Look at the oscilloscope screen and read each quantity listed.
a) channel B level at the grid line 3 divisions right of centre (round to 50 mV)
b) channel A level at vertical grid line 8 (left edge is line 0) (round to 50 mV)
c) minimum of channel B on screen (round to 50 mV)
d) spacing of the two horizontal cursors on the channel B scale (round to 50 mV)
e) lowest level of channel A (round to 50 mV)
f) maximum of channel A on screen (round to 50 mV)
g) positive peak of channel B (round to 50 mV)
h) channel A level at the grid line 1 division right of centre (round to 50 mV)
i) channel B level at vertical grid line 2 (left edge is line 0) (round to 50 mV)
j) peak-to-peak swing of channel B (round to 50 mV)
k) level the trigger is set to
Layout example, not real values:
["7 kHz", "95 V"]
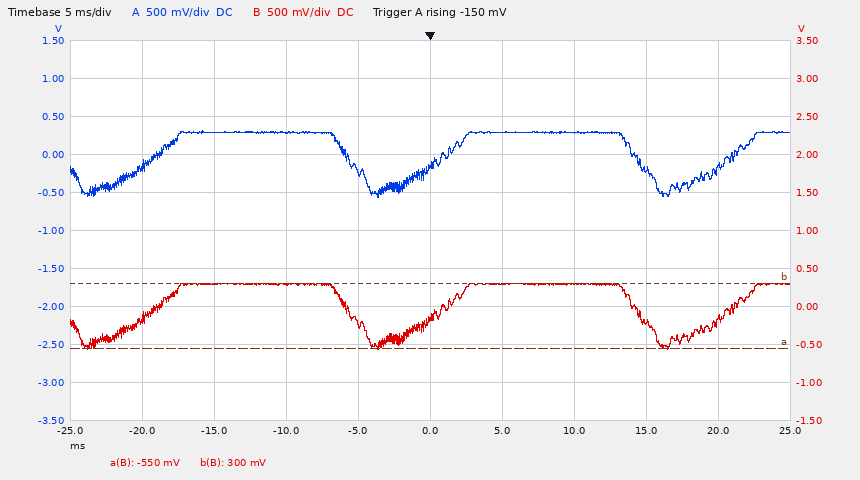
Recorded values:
["-200 mV", "-200 mV", "-550 mV", "850 mV", "-550 mV", "300 mV", "300 mV", "300 mV", "300 mV", "850 mV", "-150 mV"]
